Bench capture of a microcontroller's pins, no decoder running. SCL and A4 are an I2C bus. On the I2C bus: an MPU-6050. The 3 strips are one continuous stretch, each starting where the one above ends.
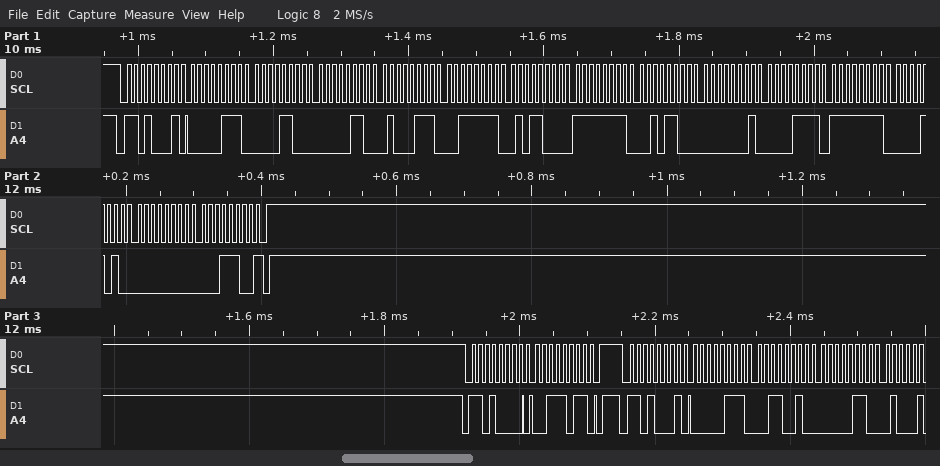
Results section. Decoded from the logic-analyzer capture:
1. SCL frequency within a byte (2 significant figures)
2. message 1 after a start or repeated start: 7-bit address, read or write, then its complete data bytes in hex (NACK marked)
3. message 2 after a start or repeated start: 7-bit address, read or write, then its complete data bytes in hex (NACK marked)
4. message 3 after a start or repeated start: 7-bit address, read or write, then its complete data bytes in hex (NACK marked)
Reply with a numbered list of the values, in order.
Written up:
1. 100 kHz
2. 0x68 read: 07 0C 06 47 3F 58 FF 2C 01 0F FF 0A 00 1C NACK
3. 0x68 write: 3B
4. 0x68 read: 07 32 06
